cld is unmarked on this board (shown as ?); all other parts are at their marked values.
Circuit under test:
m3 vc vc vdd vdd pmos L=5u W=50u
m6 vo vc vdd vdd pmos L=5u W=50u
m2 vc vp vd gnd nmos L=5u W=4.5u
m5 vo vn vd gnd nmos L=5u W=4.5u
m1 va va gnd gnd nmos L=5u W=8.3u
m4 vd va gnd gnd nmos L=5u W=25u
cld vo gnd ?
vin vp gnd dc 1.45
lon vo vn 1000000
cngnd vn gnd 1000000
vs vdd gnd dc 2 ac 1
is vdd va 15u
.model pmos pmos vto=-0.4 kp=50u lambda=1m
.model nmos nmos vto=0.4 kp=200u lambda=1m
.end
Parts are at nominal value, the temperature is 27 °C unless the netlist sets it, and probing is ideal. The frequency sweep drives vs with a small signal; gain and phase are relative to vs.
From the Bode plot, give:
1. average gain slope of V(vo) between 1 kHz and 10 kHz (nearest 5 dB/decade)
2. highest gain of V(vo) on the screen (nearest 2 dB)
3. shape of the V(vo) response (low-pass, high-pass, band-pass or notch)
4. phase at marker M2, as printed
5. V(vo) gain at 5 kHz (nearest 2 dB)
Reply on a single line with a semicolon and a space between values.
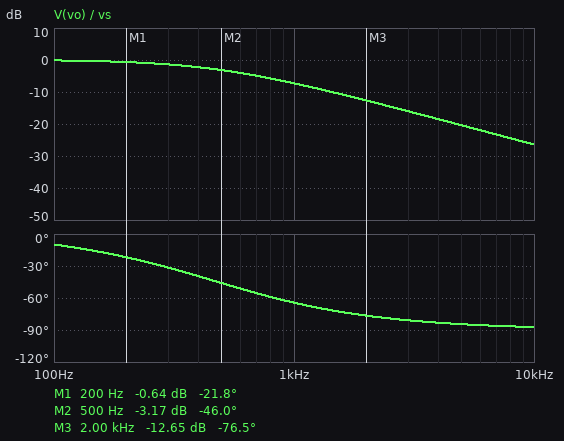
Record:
-20 dB/decade; 0 dB; low-pass; -46.0 deg; -20 dB
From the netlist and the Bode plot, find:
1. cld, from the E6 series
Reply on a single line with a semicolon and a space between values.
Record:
15 pF
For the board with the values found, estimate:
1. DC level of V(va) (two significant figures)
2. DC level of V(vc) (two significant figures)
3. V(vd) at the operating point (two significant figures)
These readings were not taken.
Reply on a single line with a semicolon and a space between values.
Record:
700 mV; 1.3 V; 550 mV
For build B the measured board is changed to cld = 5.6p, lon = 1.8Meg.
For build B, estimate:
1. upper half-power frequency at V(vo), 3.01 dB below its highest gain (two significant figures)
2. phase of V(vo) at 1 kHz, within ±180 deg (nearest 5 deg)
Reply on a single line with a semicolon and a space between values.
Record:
1.3 kHz; -40 deg
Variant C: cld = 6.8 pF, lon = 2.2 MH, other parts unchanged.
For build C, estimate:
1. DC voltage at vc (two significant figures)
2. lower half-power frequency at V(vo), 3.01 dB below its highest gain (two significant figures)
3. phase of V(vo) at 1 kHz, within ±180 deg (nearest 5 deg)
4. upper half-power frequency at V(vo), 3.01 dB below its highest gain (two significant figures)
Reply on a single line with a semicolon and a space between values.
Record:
1.3 V; 1.6 Hz; -45 deg; 1.1 kHz
